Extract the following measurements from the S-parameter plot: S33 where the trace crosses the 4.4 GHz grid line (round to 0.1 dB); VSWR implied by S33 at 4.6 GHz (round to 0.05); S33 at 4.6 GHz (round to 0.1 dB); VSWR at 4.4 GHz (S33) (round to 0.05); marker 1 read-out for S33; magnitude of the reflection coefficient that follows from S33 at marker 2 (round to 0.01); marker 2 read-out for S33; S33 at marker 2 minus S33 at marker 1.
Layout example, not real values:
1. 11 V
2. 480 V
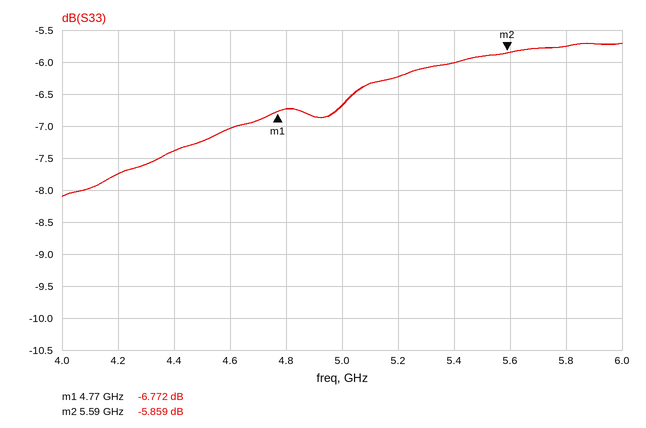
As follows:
1. -7.4 dB
2. 2.60
3. -7.0 dB
4. 2.50
5. -6.772 dB
6. 0.51
7. -5.859 dB
8. 0.913 dB
